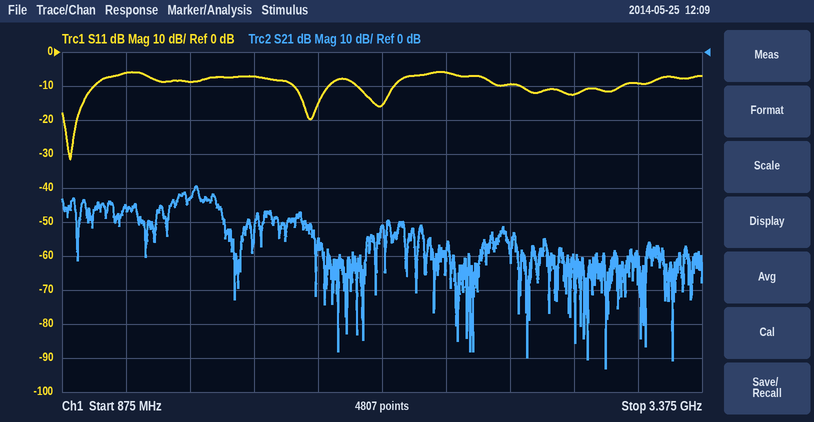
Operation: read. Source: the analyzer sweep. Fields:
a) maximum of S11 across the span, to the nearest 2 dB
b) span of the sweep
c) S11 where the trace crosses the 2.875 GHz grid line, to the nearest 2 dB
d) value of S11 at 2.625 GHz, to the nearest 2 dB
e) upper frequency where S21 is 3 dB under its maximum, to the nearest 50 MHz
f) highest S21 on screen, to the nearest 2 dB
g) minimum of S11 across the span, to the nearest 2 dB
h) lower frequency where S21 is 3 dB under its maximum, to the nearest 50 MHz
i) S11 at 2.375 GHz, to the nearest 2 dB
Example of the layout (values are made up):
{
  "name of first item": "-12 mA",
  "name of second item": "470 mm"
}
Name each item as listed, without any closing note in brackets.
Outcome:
{
  "maximum of S11 across the span, to the nearest 2 dB": "-6 dB",
  "span of the sweep": "2.5 GHz",
  "S11 where the trace crosses the 2.875 GHz grid line, to the nearest 2 dB": "-12 dB",
  "value of S11 at 2.625 GHz, to the nearest 2 dB": "-10 dB",
  "upper frequency where S21 is 3 dB under its maximum, to the nearest 50 MHz": "1.40 GHz",
  "highest S21 on screen, to the nearest 2 dB": "-40 dB",
  "minimum of S11 across the span, to the nearest 2 dB": "-32 dB",
  "lower frequency where S21 is 3 dB under its maximum, to the nearest 50 MHz": "1.40 GHz",
  "S11 at 2.375 GHz, to the nearest 2 dB": "-6 dB"
}
